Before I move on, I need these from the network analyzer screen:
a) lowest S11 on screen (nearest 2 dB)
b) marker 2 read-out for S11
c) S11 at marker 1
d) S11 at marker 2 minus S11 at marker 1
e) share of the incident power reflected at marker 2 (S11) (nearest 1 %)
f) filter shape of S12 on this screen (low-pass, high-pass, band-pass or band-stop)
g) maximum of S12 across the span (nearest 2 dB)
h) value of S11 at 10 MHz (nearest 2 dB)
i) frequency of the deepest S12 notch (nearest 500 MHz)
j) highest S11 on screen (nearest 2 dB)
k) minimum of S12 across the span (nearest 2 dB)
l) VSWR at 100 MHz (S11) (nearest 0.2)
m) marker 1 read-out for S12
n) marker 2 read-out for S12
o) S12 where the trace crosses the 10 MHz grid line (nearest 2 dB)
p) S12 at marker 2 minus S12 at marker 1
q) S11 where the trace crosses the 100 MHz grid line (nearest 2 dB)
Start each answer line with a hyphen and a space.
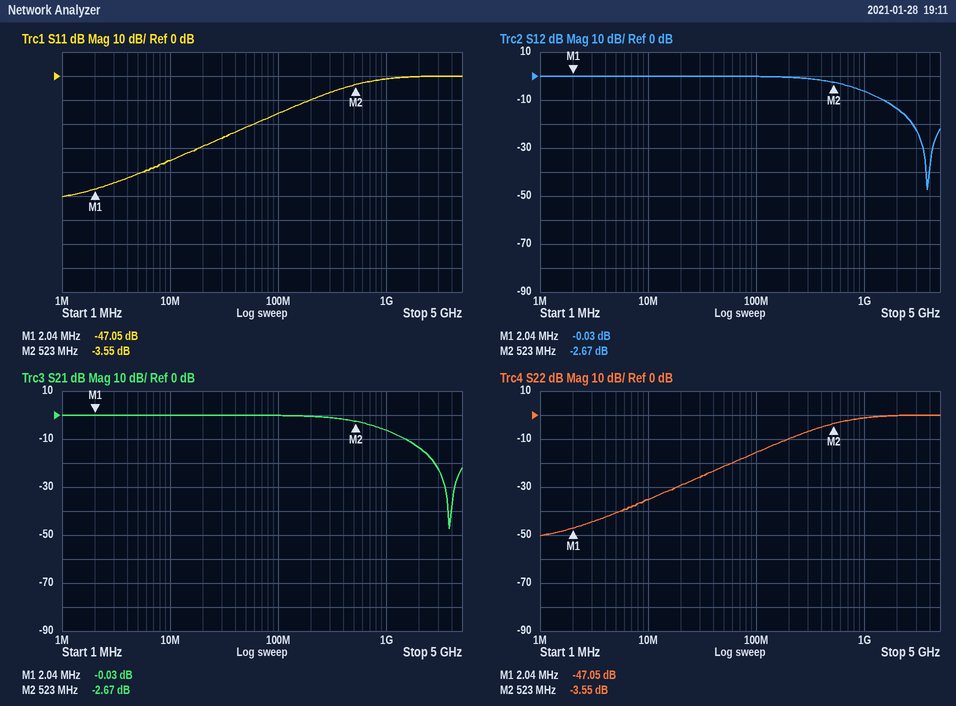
- -50 dB
- -3.55 dB
- -47.05 dB
- 43.50 dB
- 44 %
- low-pass
- 0 dB
- -36 dB
- 4.0 GHz
- 0 dB
- -48 dB
- 1.4
- -0.03 dB
- -2.67 dB
- 0 dB
- -2.64 dB
- -16 dB
